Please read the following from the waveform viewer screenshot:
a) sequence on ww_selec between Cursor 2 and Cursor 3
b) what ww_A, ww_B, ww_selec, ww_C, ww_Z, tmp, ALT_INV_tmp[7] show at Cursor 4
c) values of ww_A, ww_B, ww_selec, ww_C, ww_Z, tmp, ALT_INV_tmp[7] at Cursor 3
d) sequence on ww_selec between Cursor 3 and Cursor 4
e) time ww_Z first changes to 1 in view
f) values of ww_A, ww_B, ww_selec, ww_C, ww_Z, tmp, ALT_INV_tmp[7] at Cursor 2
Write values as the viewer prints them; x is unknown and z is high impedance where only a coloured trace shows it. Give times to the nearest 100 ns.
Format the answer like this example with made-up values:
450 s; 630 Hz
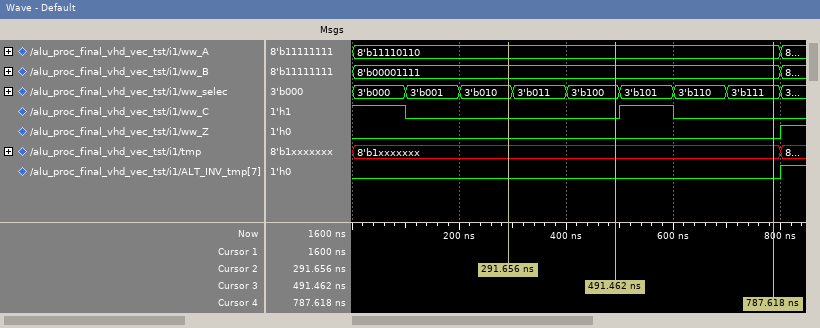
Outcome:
3'b010, 3'b011, 3'b100; ww_A=8'b11110110, ww_B=8'b00001111, ww_selec=3'b111, ww_C=0, ww_Z=0, tmp=8'b1xxxxxxx, ALT_INV_tmp[7]=0; ww_A=8'b11110110, ww_B=8'b00001111, ww_selec=3'b100, ww_C=0, ww_Z=0, tmp=8'b1xxxxxxx, ALT_INV_tmp[7]=0; 3'b100, 3'b101, 3'b110, 3'b111; 800 ns; ww_A=8'b11110110, ww_B=8'b00001111, ww_selec=3'b010, ww_C=0, ww_Z=0, tmp=8'b1xxxxxxx, ALT_INV_tmp[7]=0
